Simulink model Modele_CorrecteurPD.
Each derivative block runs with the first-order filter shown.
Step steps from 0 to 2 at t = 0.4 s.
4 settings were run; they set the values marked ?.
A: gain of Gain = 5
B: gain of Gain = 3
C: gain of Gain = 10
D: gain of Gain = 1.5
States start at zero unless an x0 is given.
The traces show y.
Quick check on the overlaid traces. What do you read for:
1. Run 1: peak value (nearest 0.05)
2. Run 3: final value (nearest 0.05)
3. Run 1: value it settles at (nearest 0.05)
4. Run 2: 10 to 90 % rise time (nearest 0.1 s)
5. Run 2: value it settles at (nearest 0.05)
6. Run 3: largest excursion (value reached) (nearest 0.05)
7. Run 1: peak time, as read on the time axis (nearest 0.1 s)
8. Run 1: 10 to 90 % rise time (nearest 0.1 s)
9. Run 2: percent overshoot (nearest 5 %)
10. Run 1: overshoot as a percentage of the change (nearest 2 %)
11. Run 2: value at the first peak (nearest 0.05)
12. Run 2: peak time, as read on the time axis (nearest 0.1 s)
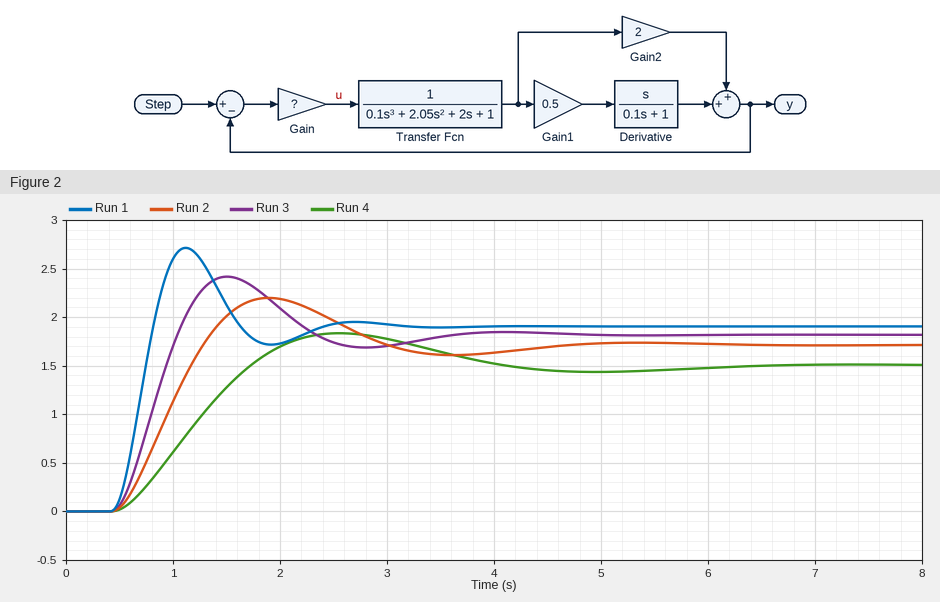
2.70
1.80
1.90
0.6 s
1.70
2.40
1.1 s
0.3 s
30 %
42 %
2.20
1.9 s
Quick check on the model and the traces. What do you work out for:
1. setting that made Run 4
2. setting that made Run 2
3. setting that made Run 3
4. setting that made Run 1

D
B
A
C
